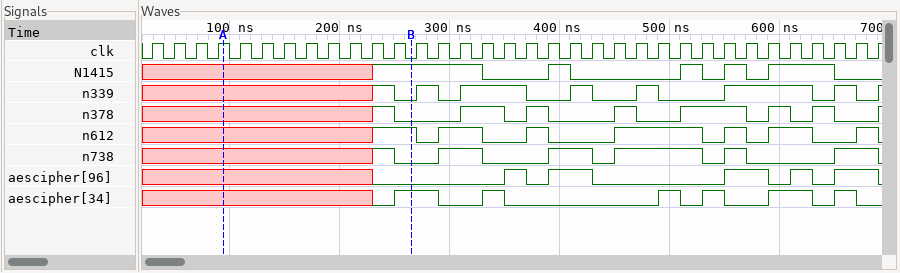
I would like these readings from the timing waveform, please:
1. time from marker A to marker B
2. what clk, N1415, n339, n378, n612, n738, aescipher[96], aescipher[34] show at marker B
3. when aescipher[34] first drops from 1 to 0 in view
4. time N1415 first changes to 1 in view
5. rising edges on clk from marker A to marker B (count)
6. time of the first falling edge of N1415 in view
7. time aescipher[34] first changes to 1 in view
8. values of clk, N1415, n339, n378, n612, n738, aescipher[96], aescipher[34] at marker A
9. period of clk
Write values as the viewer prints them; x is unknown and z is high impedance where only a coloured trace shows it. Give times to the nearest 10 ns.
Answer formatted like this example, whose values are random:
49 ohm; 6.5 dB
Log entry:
170 ns; clk=0, N1415=1, n339=0, n378=0, n612=1, n738=0, aescipher[96]=0, aescipher[34]=1; 290 ns; 230 ns; 8; 330 ns; 250 ns; clk=1, N1415=x, n339=x, n378=x, n612=x, n738=x, aescipher[96]=x, aescipher[34]=x; 20 ns
